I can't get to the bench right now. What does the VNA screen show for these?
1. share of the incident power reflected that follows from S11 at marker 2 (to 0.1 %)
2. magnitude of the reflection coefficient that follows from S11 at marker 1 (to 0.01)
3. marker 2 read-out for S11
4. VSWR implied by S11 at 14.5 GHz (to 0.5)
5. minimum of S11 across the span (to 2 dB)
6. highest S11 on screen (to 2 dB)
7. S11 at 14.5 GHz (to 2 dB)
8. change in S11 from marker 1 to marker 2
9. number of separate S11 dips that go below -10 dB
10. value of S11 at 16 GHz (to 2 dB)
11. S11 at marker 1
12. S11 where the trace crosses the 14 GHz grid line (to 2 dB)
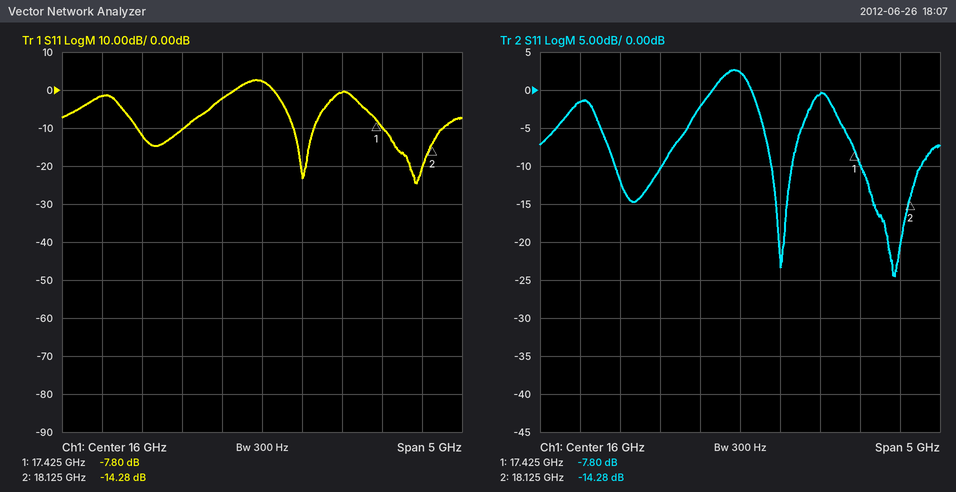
3.7 %
0.41
-14.28 dB
1.5
-24 dB
2 dB
-12 dB
-6.48 dB
3
2 dB
-7.80 dB
-2 dB
